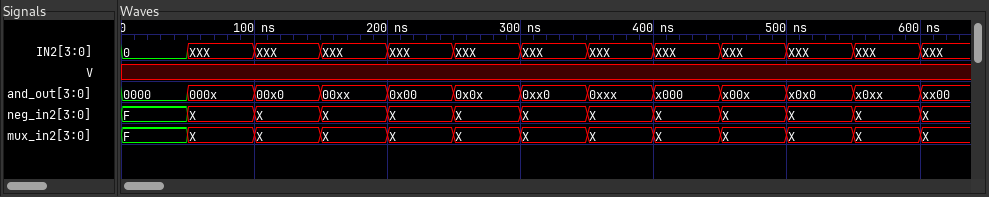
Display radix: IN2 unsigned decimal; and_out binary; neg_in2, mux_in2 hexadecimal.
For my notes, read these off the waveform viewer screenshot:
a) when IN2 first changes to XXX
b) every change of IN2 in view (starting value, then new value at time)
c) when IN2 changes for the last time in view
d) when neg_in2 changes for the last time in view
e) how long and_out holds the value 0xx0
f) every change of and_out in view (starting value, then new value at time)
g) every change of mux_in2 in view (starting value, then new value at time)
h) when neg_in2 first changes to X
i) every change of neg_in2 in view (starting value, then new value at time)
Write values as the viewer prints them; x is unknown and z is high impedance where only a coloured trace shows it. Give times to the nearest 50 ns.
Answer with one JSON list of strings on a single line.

["50 ns", "0, XXX at 50 ns, XXX at 100 ns, XXX at 150 ns, XXX at 200 ns, XXX at 250 ns, XXX at 300 ns, XXX at 350 ns, XXX at 400 ns, XXX at 450 ns, XXX at 500 ns, XXX at 550 ns, XXX at 600 ns", "600 ns", "600 ns", "50 ns", "0000, 000x at 50 ns, 00x0 at 100 ns, 00xx at 150 ns, 0x00 at 200 ns, 0x0x at 250 ns, 0xx0 at 300 ns, 0xxx at 350 ns, x000 at 400 ns, x00x at 450 ns, x0x0 at 500 ns, x0xx at 550 ns, xx00 at 600 ns", "F, X at 50 ns, X at 100 ns, X at 150 ns, X at 200 ns, X at 250 ns, X at 300 ns, X at 350 ns, X at 400 ns, X at 450 ns, X at 500 ns, X at 550 ns, X at 600 ns", "50 ns", "F, X at 50 ns, X at 100 ns, X at 150 ns, X at 200 ns, X at 250 ns, X at 300 ns, X at 350 ns, X at 400 ns, X at 450 ns, X at 500 ns, X at 550 ns, X at 600 ns"]
